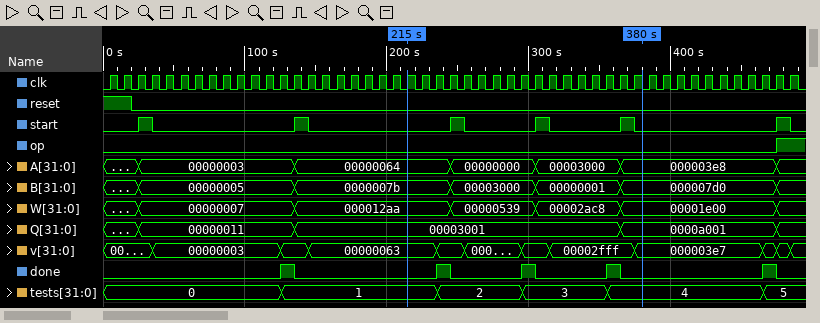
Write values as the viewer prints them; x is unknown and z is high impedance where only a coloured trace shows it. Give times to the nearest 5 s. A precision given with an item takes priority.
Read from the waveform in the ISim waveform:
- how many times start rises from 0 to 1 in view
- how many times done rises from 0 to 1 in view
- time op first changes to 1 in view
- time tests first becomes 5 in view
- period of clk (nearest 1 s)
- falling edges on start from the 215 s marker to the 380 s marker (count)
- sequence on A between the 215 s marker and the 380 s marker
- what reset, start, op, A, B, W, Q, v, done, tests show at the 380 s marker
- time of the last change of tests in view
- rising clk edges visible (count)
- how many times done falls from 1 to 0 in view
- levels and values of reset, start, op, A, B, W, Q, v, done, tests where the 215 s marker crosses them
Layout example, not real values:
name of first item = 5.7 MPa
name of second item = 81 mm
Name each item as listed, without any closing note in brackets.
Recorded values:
how many times start rises from 0 to 1 in view = 6
how many times done rises from 0 to 1 in view = 5
time op first changes to 1 in view = 475 s
time tests first becomes 5 in view = 465 s
period of clk = 10 s
falling edges on start from the 215 s marker to the 380 s marker = 3
sequence on A between the 215 s marker and the 380 s marker = 00000064, 00000000, 00003000, 000003e8
what reset, start, op, A, B, W, Q, v, done, tests show at the 380 s marker = reset=0, start=0, op=0, A=000003e8, B=000007d0, W=00001e00, Q=0000a001, v=000003e7, done=0, tests=4
time of the last change of tests in view = 465 s
rising clk edges visible = 49
how many times done falls from 1 to 0 in view = 5
levels and values of reset, start, op, A, B, W, Q, v, done, tests where the 215 s marker crosses them = reset=0, start=0, op=0, A=00000064, B=0000007b, W=000012aa, Q=00003001, v=00000063, done=0, tests=1
